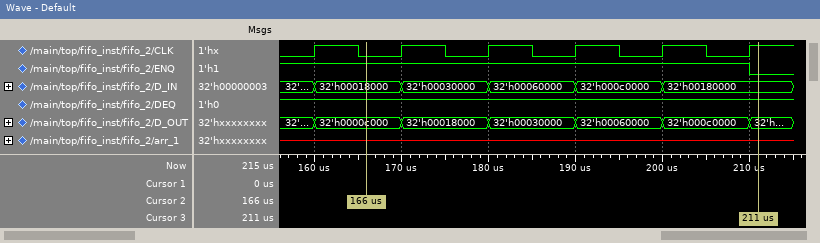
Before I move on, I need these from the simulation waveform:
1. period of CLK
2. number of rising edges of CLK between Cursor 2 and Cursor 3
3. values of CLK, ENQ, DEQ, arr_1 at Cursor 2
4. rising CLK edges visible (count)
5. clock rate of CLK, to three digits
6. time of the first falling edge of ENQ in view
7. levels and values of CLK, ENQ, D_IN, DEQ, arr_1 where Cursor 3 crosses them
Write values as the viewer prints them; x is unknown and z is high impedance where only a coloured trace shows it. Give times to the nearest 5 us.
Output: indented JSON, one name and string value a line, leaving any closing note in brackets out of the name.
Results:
{
  "period of CLK": "10 us",
  "number of rising edges of CLK between Cursor 2 and Cursor 3": "5",
  "values of CLK, ENQ, DEQ, arr_1 at Cursor 2": "CLK=0, ENQ=1, DEQ=1, arr_1=x",
  "rising CLK edges visible": "6",
  "clock rate of CLK, to three digits": "100 kHz",
  "time of the first falling edge of ENQ in view": "210 us",
  "levels and values of CLK, ENQ, D_IN, DEQ, arr_1 where Cursor 3 crosses them": "CLK=1, ENQ=0, D_IN=32'h00180000, DEQ=1, arr_1=x"
}
